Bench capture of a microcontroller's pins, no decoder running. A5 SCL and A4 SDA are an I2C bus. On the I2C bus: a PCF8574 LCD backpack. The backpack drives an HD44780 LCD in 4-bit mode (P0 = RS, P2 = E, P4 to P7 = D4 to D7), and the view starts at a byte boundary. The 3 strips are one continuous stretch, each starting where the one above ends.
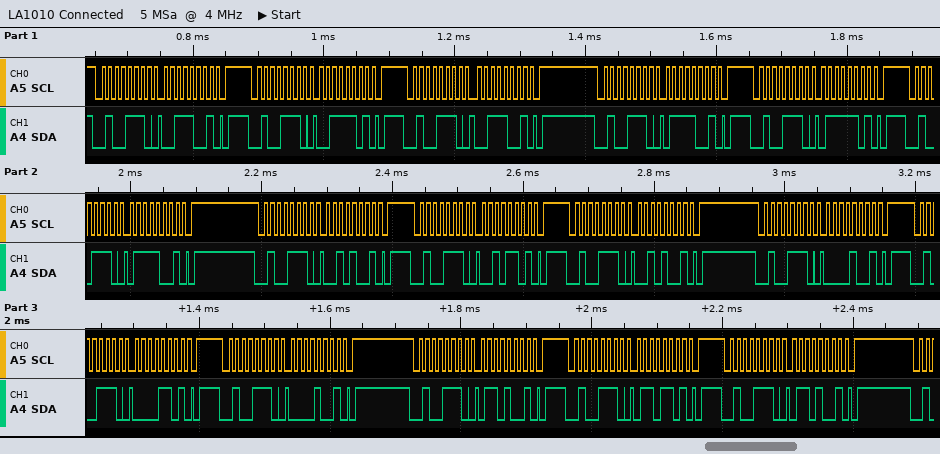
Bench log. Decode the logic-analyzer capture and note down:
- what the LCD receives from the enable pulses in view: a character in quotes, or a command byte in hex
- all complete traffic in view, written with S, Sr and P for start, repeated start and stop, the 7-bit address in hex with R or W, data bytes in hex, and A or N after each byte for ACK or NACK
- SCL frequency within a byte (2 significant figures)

'7' ' '
S 27W A 39 A P S 27W A 3D A P S 27W A 39 A P S 27W A 79 A P S 27W A 7D A P S 27W A 79 A P S 27W A 29 A P S 27W A 2D A P S 27W A 29 A P S 27W A 09 A P S 27W A 0D A P S 27W A 09 A P S 27W A 69 A P S 27W A 6D A P S 27W A 69 A P
100 kHz
